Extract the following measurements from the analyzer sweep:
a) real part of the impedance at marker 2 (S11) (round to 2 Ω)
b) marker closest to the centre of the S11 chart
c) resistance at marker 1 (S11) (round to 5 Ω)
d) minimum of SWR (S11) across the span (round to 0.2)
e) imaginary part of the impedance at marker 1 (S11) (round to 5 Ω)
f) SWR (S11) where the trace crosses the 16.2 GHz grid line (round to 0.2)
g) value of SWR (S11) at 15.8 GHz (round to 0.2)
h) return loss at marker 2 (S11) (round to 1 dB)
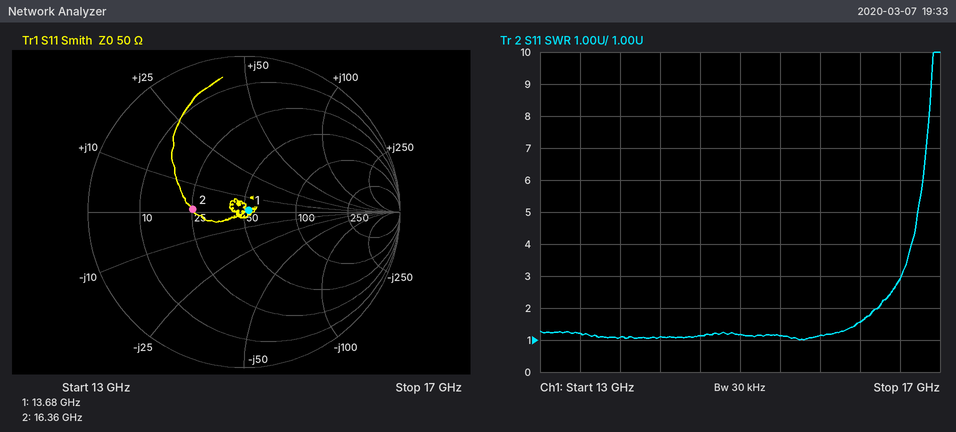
26 Ω
marker 1
55 Ω
1.0
0 Ω
1.6
1.2
10 dB
